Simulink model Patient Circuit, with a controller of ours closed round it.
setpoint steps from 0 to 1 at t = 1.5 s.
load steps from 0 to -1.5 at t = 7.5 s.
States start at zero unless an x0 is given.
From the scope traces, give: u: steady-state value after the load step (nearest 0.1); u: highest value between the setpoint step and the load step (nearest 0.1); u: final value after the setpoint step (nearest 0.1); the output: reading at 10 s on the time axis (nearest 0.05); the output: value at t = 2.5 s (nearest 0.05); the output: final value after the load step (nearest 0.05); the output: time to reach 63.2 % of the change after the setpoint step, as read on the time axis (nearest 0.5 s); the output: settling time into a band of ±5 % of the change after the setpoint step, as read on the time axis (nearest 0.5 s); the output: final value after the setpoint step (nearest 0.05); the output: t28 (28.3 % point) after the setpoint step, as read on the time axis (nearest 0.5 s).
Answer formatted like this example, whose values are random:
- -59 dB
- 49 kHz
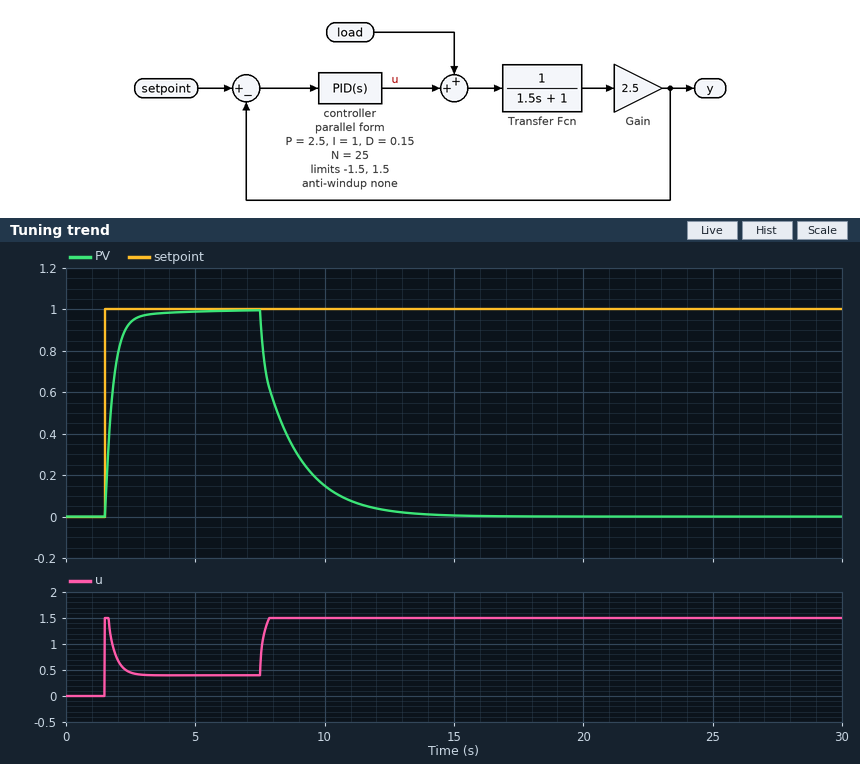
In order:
- 1.5
- 1.5
- 0.4
- 0.15
- 0.95
- 0.00
- 2.0 s
- 2.5 s
- 1.00
- 1.5 s
